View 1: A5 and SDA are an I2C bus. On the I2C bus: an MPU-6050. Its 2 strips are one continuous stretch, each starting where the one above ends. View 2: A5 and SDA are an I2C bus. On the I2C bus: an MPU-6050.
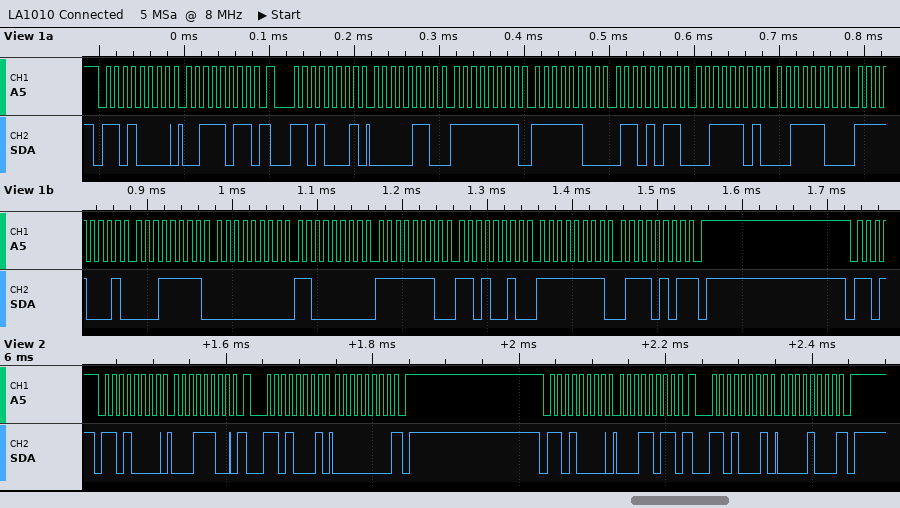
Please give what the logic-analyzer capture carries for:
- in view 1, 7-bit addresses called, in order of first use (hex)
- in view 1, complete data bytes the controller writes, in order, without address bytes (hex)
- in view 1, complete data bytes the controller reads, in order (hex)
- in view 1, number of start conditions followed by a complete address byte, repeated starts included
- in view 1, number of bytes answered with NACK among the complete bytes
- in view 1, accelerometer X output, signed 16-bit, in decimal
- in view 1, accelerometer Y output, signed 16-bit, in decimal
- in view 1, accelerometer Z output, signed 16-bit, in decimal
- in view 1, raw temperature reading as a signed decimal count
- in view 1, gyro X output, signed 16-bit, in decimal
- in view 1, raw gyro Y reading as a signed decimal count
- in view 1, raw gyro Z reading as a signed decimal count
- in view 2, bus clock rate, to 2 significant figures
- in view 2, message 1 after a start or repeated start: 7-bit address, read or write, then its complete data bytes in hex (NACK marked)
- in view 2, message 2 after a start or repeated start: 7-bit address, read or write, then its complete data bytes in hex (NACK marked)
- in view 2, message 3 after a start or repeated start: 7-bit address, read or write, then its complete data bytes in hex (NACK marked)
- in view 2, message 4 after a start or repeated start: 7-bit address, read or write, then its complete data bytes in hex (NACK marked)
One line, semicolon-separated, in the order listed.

0x68; 3B; 06 FF FC 6B 3D 3C F1 1F 00 C0 FE D2 FF 75; 2; 1; 1791; -917; 15676; -3809; 192; -302; -139; 100 kHz; 0x68 write: 1C; 0x68 read: 00 NACK; 0x68 write: 1B; 0x68 read: 08 NACK
